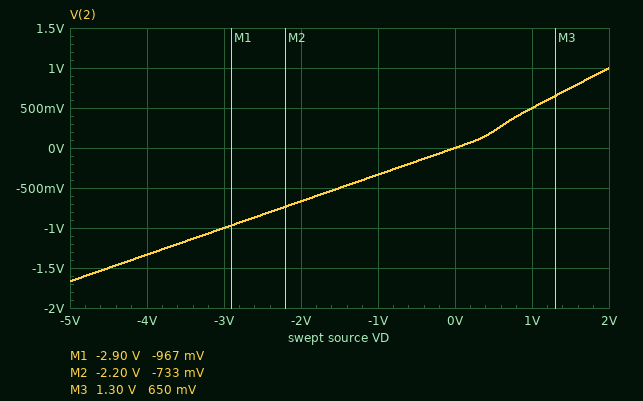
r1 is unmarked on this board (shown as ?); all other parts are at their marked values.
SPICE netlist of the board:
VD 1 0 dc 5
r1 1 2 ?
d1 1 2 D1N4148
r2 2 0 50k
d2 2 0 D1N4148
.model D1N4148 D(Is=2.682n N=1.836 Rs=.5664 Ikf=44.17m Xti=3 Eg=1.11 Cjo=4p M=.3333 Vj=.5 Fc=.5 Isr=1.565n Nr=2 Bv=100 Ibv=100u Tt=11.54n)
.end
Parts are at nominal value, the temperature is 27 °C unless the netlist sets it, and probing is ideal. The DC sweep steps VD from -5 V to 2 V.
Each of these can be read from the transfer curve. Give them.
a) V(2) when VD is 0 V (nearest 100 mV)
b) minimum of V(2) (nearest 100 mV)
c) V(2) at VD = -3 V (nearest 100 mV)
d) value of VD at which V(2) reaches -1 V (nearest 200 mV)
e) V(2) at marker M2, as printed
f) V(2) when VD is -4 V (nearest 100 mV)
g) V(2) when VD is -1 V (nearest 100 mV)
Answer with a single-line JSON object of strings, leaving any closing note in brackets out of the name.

{"V(2) when VD is 0 V": "0 V", "minimum of V(2)": "-1.7 V", "V(2) at VD = -3 V": "-1.0 V", "value of VD at which V(2) reaches -1 V": "-3.0 V", "V(2) at marker M2, as printed": "-733 mV", "V(2) when VD is -4 V": "-1.3 V", "V(2) when VD is -1 V": "-300 mV"}
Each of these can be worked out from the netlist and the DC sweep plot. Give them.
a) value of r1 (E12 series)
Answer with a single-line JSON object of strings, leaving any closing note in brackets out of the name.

{"value of r1": "100 kΩ"}
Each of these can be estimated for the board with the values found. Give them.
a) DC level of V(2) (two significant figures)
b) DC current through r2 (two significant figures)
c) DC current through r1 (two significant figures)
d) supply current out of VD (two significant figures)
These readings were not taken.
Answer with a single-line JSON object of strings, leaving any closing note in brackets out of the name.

{"DC level of V(2)": "2.5 V", "DC current through r2": "50 µA", "DC current through r1": "25 µA", "supply current out of VD": "2.4 A"}
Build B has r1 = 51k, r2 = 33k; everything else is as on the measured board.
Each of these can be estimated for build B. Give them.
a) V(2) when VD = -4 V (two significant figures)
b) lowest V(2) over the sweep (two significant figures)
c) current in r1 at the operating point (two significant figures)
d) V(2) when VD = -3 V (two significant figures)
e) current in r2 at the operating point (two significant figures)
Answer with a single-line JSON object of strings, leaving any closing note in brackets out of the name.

{"V(2) when VD = -4 V": "-1.6 V", "lowest V(2) over the sweep": "-2.0 V", "current in r1 at the operating point": "49 µA", "V(2) when VD = -3 V": "-1.2 V", "current in r2 at the operating point": "76 µA"}
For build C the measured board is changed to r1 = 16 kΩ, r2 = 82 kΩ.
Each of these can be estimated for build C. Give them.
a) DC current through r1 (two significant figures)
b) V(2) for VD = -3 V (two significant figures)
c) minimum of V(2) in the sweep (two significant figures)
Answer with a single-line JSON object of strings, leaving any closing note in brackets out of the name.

{"DC current through r1": "160 µA", "V(2) for VD = -3 V": "-2.5 V", "minimum of V(2) in the sweep": "-4.2 V"}
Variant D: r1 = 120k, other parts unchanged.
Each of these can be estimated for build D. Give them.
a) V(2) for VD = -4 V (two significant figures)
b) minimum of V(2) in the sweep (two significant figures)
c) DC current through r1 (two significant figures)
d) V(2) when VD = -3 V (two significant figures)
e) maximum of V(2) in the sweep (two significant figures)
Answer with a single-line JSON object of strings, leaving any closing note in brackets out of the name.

{"V(2) for VD = -4 V": "-1.2 V", "minimum of V(2) in the sweep": "-1.5 V", "DC current through r1": "21 µA", "V(2) when VD = -3 V": "-880 mV", "maximum of V(2) in the sweep": "1.0 V"}
